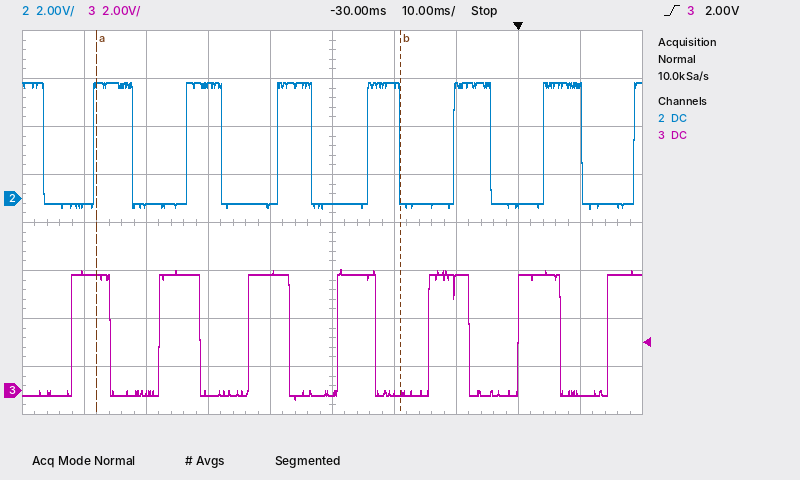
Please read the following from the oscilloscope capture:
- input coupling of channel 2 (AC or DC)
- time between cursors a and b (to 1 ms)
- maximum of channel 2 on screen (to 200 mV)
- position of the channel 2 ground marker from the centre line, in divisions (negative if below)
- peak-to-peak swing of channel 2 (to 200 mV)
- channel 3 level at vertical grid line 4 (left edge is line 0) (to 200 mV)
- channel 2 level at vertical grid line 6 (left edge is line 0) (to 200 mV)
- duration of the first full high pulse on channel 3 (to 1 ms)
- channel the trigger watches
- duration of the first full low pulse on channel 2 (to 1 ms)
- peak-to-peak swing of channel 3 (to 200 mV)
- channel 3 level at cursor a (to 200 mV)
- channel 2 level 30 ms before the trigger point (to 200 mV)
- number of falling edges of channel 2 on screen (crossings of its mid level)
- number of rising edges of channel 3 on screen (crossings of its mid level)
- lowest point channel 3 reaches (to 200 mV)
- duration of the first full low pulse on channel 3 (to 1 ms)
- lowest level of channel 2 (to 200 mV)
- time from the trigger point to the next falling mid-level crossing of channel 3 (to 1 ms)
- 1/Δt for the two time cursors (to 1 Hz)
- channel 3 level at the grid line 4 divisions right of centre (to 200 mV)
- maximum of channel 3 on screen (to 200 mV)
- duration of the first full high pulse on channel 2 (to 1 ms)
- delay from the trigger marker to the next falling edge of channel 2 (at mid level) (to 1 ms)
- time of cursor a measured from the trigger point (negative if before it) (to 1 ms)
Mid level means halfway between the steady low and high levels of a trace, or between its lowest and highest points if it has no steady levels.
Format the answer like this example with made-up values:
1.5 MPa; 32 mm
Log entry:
DC; 49 ms; 4.8 V; +0.5 div; 5.2 V; 4.8 V; 4.8 V; 6 ms; channel 3; 8 ms; 5.4 V; 4.8 V; -200 mV; 7; 7; -400 mV; 8 ms; -400 mV; 7 ms; 20 Hz; -200 mV; 5.0 V; 6 ms; 10 ms; -68 ms
